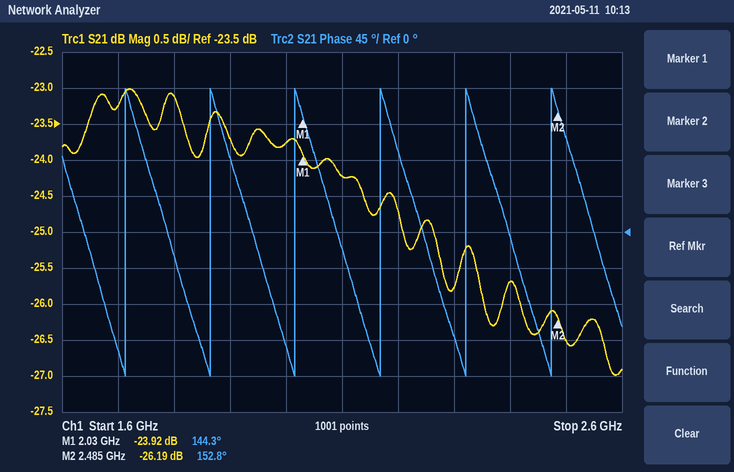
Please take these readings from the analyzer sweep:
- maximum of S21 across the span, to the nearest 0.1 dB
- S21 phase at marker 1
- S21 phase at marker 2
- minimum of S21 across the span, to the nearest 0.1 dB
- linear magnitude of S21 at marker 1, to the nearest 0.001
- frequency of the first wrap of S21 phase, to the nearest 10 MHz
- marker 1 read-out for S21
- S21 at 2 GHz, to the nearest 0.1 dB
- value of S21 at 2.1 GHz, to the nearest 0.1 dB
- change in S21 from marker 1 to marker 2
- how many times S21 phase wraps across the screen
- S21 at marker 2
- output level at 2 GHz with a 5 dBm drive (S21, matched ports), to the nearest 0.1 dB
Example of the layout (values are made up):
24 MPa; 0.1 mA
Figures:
-23.0 dB; 144.3°; 152.8°; -27.0 dB; 0.064; 1.71 GHz; -23.92 dB; -23.8 dB; -24.2 dB; -2.27 dB; 6; -26.19 dB; -18.8 dBm
